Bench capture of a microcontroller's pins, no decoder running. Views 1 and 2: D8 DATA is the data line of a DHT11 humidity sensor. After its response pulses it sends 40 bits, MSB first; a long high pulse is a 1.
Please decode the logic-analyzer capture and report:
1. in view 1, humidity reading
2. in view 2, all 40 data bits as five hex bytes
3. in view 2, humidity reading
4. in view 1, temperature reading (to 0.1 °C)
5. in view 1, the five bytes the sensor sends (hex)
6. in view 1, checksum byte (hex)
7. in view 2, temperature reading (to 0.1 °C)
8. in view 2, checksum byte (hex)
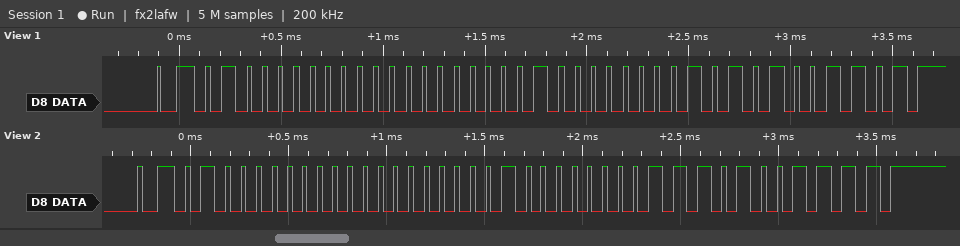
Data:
64 %
40 00 08 07 4F
64 %
8.5 °C
40 00 08 05 4D
0x4D
8.7 °C
0x4F
